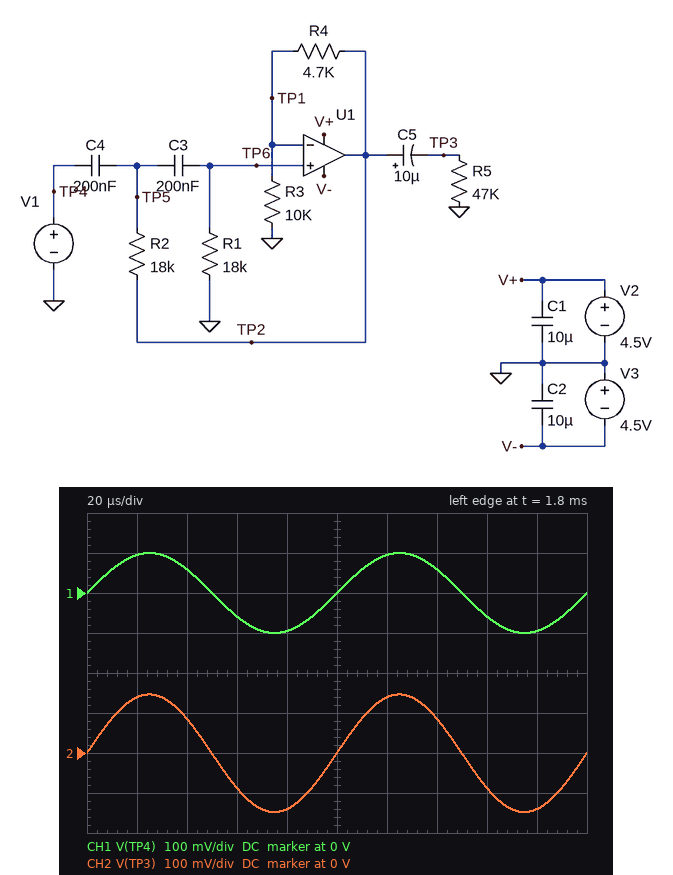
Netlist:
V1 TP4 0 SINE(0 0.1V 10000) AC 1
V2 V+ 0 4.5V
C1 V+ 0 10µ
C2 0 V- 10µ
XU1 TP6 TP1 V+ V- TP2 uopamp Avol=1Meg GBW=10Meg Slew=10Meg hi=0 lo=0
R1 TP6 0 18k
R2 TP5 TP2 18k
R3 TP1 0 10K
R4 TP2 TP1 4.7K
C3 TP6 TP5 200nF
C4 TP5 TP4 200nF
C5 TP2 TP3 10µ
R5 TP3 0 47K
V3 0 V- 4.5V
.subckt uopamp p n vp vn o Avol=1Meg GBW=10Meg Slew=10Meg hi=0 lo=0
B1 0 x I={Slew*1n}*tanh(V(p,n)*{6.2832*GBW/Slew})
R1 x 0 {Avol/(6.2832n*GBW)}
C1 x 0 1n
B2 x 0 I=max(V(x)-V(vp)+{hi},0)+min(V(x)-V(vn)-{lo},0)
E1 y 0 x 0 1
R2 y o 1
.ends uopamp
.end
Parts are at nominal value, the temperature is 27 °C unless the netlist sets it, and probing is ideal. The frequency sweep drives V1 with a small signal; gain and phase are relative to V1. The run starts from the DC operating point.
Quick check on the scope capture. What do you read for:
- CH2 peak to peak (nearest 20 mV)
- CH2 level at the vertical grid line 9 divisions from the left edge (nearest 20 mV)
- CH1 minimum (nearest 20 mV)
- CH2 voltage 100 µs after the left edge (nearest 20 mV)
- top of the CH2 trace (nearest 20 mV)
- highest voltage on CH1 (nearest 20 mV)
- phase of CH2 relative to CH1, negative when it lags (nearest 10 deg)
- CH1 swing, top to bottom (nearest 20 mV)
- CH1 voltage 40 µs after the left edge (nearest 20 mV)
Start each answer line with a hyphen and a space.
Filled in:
- 300 mV
- -140 mV
- -100 mV
- 0 V
- 140 mV
- 100 mV
- 0 deg
- 200 mV
- 60 mV
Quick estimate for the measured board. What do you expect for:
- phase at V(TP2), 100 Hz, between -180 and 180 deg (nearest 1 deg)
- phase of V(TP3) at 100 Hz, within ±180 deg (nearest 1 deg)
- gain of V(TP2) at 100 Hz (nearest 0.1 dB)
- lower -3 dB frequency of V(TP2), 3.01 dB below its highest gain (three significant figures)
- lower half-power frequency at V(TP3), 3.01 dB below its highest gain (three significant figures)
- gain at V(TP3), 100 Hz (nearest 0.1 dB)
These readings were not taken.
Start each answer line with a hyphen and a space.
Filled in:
- 40 deg
- 40 deg
- 2.9 dB
- 48.1 Hz
- 48.1 Hz
- 2.9 dB
